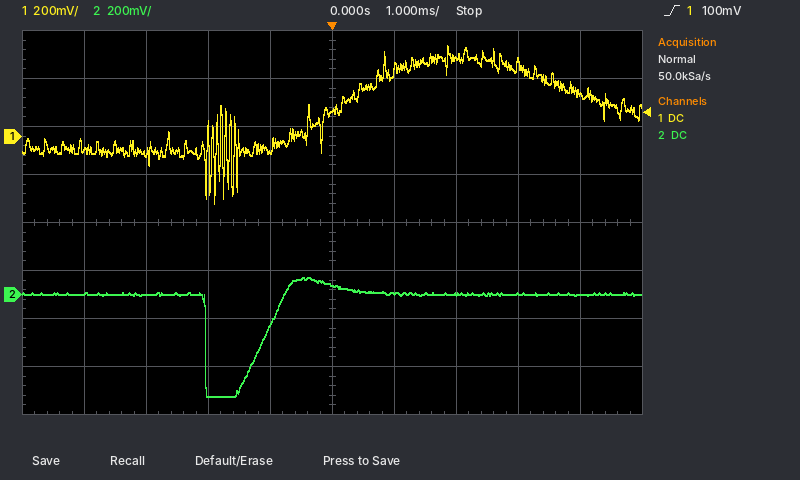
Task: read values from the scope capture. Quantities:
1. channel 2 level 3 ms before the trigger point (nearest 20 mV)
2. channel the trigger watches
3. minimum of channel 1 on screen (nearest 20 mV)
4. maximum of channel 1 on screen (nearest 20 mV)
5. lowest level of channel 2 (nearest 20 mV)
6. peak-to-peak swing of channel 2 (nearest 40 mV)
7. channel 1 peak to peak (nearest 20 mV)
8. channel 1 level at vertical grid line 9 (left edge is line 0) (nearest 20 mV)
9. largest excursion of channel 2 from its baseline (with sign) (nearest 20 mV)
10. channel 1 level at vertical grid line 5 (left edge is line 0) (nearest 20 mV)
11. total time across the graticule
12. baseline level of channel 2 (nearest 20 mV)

0 mV
channel 1
-280 mV
380 mV
-420 mV
480 mV
660 mV
180 mV
-420 mV
100 mV
10 ms
0 mV
